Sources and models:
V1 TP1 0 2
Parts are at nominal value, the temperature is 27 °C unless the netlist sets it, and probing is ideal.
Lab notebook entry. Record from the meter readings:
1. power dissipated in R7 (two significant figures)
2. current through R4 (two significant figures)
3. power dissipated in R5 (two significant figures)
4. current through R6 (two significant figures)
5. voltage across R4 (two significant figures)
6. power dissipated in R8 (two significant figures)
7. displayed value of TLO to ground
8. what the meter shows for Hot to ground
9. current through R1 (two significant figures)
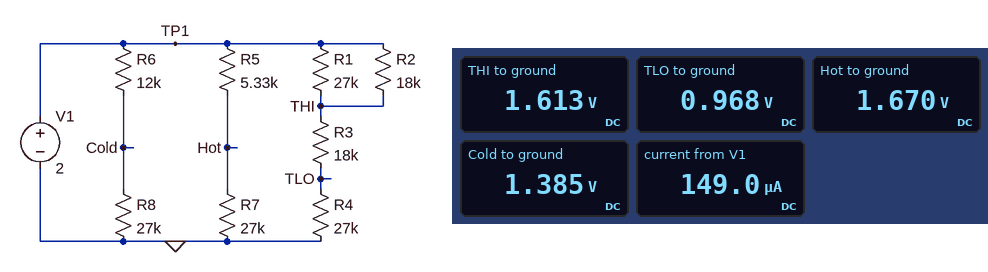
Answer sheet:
100 µW
36 µA
20 µW
51 µA
970 mV
71 µW
0.968 V
1.670 V
14 µA
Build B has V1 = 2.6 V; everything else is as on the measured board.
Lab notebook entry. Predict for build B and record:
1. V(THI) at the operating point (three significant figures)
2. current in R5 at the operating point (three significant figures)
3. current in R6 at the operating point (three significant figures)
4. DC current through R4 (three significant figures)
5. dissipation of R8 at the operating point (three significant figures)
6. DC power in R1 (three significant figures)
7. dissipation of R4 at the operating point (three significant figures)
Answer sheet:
2.10 V
80.4 µA
66.7 µA
46.6 µA
120 µW
9.38 µW
58.6 µW
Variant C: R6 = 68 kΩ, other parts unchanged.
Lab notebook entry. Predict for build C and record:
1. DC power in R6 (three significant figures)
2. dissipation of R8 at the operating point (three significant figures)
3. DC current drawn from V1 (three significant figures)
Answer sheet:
30.1 µW
12.0 µW
119 µA
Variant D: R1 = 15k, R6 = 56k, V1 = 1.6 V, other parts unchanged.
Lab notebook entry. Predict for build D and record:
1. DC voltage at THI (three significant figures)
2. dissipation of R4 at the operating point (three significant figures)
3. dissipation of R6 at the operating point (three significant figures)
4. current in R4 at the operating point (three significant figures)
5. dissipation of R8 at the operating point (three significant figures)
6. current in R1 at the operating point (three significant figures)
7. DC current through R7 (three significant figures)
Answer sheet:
1.35 V
24.4 µW
20.8 µW
30.1 µA
10.0 µW
16.4 µA
49.5 µA
